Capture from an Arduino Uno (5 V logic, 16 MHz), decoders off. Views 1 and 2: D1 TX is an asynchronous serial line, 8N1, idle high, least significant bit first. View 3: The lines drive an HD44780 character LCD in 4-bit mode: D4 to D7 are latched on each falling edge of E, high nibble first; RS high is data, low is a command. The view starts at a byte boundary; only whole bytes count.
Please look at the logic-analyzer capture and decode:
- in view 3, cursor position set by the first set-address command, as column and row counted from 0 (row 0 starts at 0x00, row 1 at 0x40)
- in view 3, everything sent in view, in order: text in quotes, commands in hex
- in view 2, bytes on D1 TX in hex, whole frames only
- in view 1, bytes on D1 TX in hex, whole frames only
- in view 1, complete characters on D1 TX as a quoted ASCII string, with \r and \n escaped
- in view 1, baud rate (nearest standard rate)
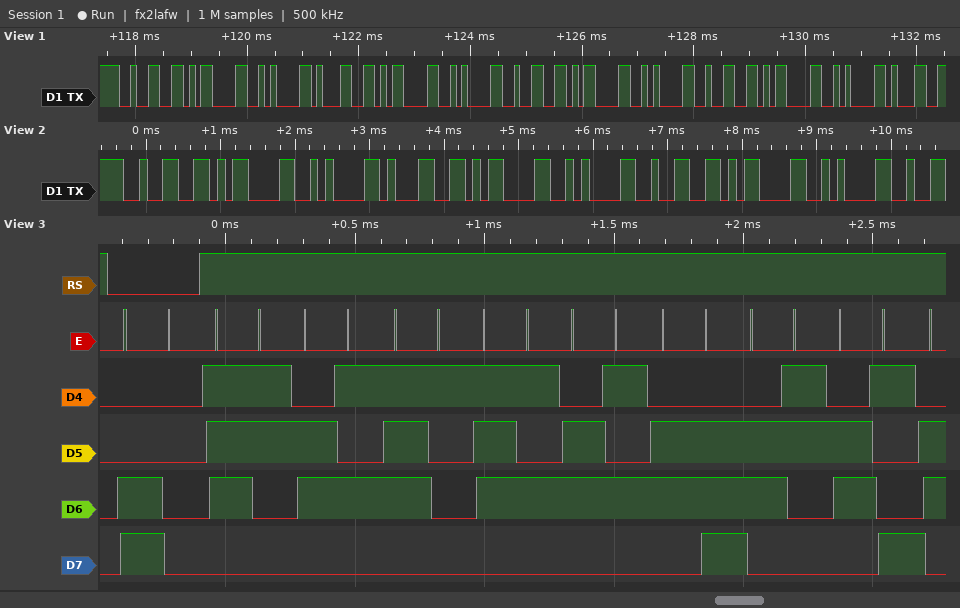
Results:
column 0, row 1
0xC0 "sequenci"
0x32 0x0D 0x0A 0x31 0x0D 0x0A 0x32 0x0D 0x0A
32 0D 0A 31 0D 0A 32 0D 0A 32 0D 0A 31
"2\r\n1\r\n2\r\n2\r\n1"
9600 baud
